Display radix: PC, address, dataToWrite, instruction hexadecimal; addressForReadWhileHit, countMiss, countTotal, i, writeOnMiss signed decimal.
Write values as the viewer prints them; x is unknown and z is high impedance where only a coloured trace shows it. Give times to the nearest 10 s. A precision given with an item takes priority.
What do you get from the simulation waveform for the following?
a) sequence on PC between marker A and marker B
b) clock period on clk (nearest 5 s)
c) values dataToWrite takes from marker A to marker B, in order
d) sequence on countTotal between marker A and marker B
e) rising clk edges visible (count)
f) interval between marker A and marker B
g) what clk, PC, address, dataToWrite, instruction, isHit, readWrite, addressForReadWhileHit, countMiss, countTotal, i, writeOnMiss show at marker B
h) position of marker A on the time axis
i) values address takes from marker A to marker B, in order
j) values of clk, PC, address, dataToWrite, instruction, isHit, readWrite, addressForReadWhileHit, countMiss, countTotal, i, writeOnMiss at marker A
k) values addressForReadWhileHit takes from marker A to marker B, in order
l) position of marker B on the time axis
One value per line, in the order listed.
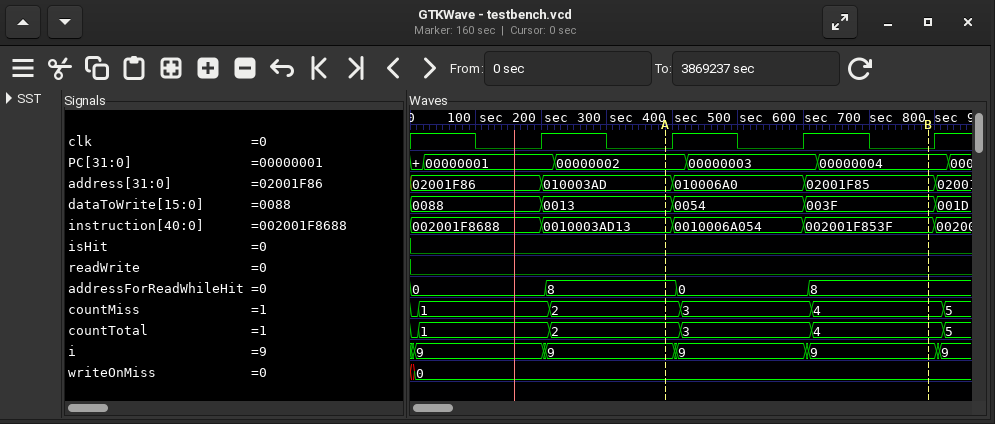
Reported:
00000002, 00000003, 00000004
200 s
0013, 0054, 003F
2, 3, 4
4
400 s
clk=0, PC=00000004, address=02001F85, dataToWrite=003F, instruction=002001F853F, isHit=0, readWrite=0, addressForReadWhileHit=8, countMiss=4, countTotal=4, i=9, writeOnMiss=0
390 s
010003AD, 010006A0, 02001F85
clk=0, PC=00000002, address=010003AD, dataToWrite=0013, instruction=0010003AD13, isHit=0, readWrite=0, addressForReadWhileHit=8, countMiss=2, countTotal=2, i=9, writeOnMiss=0
8, 0, 8
790 s
